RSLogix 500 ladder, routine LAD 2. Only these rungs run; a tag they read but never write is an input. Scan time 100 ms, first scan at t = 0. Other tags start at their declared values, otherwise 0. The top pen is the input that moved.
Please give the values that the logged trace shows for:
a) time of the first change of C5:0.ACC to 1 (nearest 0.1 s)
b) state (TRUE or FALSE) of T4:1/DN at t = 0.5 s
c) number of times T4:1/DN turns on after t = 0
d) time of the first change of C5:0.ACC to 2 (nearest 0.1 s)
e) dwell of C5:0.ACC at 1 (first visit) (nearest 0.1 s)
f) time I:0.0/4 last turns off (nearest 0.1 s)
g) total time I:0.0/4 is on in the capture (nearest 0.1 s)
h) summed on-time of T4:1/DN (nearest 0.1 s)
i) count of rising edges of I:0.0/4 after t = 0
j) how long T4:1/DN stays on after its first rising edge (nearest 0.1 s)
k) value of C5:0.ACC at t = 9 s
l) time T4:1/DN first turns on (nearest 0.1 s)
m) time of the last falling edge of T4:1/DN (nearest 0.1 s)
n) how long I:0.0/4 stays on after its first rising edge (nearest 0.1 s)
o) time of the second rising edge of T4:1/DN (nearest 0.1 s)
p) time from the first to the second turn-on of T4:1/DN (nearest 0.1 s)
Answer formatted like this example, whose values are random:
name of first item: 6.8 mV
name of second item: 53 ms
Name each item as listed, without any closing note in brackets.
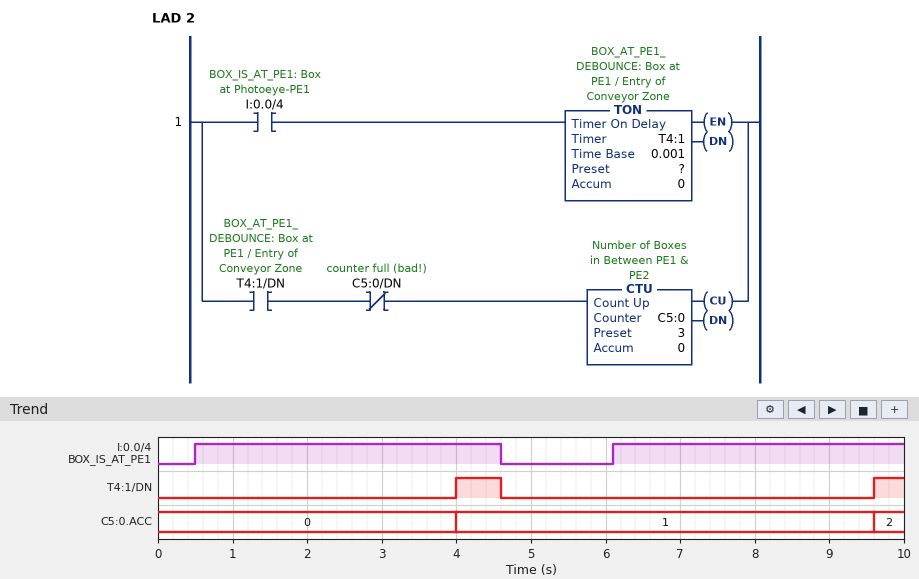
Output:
time of the first change of C5:0.ACC to 1: 4.0 s
state (TRUE or FALSE) of T4:1/DN at t = 0.5 s: FALSE
number of times T4:1/DN turns on after t = 0: 2
time of the first change of C5:0.ACC to 2: 9.6 s
dwell of C5:0.ACC at 1 (first visit): 5.6 s
time I:0.0/4 last turns off: 4.6 s
total time I:0.0/4 is on in the capture: 8.0 s
summed on-time of T4:1/DN: 1.0 s
count of rising edges of I:0.0/4 after t = 0: 2
how long T4:1/DN stays on after its first rising edge: 0.6 s
value of C5:0.ACC at t = 9 s: 1
time T4:1/DN first turns on: 4.0 s
time of the last falling edge of T4:1/DN: 4.6 s
how long I:0.0/4 stays on after its first rising edge: 4.1 s
time of the second rising edge of T4:1/DN: 9.6 s
time from the first to the second turn-on of T4:1/DN: 5.6 s
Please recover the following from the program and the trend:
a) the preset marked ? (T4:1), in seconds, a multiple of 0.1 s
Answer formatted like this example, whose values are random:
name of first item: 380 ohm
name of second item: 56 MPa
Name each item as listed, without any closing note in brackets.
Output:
the preset marked ? (T4:1), in seconds, a multiple of 0.1 s: 3.5 s
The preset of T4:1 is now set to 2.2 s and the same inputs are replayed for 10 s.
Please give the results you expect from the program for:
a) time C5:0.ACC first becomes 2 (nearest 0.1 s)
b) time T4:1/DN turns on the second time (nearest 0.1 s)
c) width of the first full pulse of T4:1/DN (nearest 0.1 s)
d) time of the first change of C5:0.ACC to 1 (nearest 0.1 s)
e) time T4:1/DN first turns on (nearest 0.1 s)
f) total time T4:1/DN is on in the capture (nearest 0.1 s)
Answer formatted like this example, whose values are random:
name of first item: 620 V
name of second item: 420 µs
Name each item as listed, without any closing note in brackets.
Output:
time C5:0.ACC first becomes 2: 8.3 s
time T4:1/DN turns on the second time: 8.3 s
width of the first full pulse of T4:1/DN: 1.9 s
time of the first change of C5:0.ACC to 1: 2.7 s
time T4:1/DN first turns on: 2.7 s
total time T4:1/DN is on in the capture: 3.6 s
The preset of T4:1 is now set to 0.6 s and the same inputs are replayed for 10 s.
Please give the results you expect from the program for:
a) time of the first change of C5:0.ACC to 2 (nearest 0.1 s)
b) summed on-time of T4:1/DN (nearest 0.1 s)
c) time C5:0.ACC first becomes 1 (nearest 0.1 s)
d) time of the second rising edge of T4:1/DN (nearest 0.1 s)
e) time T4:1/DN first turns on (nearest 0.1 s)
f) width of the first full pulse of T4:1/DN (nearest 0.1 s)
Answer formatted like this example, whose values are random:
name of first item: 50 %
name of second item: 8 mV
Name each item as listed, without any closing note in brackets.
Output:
time of the first change of C5:0.ACC to 2: 6.7 s
summed on-time of T4:1/DN: 6.8 s
time C5:0.ACC first becomes 1: 1.1 s
time of the second rising edge of T4:1/DN: 6.7 s
time T4:1/DN first turns on: 1.1 s
width of the first full pulse of T4:1/DN: 3.5 s
